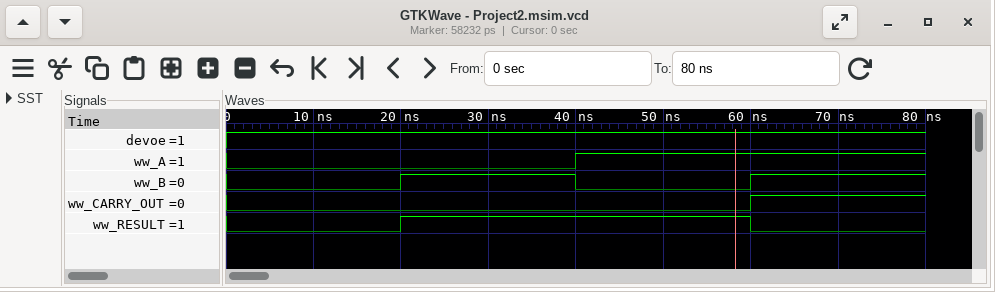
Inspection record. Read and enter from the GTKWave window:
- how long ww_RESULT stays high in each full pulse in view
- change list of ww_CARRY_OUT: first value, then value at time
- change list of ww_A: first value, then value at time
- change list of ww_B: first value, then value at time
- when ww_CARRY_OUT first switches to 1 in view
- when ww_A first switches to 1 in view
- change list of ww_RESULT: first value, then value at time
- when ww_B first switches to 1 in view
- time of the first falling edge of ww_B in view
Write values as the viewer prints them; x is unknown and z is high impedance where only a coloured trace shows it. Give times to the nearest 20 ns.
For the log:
40 ns
0, 1 at 60 ns
0, 1 at 40 ns
0, 1 at 20 ns, 0 at 40 ns, 1 at 60 ns
60 ns
40 ns
0, 1 at 20 ns, 0 at 60 ns
20 ns
40 ns
